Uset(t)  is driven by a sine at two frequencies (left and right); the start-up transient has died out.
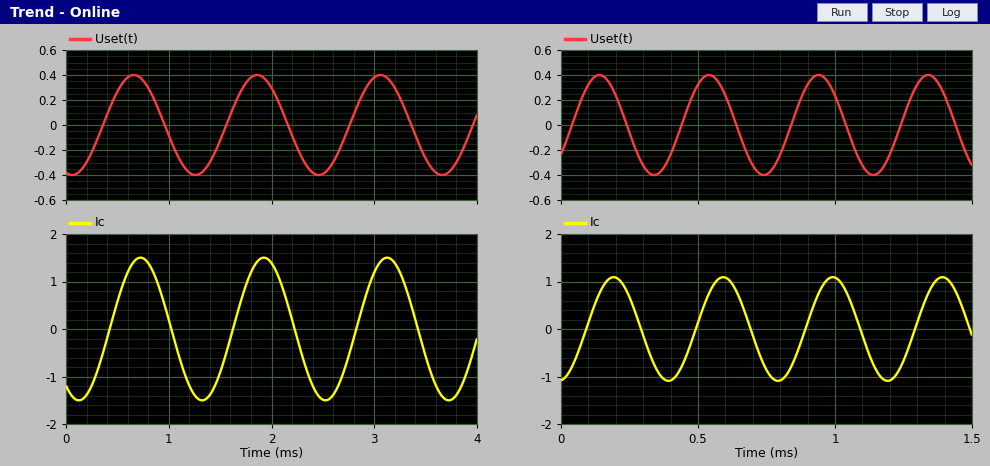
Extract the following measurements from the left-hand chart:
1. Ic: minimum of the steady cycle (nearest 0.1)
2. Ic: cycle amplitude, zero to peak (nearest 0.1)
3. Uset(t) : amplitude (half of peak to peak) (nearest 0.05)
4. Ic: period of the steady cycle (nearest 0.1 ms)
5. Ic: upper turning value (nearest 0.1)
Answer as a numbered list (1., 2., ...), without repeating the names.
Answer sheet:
1. -1.5
2. 1.5
3. 0.40
4. 1.2 ms
5. 1.5
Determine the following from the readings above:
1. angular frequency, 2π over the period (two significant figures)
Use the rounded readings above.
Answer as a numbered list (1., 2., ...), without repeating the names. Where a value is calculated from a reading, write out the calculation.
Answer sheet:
1. 2π / 1.2 = 5.2 rad/ms
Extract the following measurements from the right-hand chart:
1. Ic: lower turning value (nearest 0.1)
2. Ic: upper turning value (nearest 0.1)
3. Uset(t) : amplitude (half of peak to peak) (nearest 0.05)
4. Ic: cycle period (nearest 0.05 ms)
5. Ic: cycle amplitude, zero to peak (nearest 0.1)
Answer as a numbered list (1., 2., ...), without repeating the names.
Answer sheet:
1. -1.1
2. 1.1
3. 0.40
4. 0.40 ms
5. 1.1
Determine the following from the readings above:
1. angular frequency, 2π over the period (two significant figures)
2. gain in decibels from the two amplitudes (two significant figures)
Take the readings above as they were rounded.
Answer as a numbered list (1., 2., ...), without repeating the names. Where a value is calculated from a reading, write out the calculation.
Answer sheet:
1. 2π / 0.4 = 16 rad/ms
2. 20 log10(1.1 / 0.4) = 8.8 dB
